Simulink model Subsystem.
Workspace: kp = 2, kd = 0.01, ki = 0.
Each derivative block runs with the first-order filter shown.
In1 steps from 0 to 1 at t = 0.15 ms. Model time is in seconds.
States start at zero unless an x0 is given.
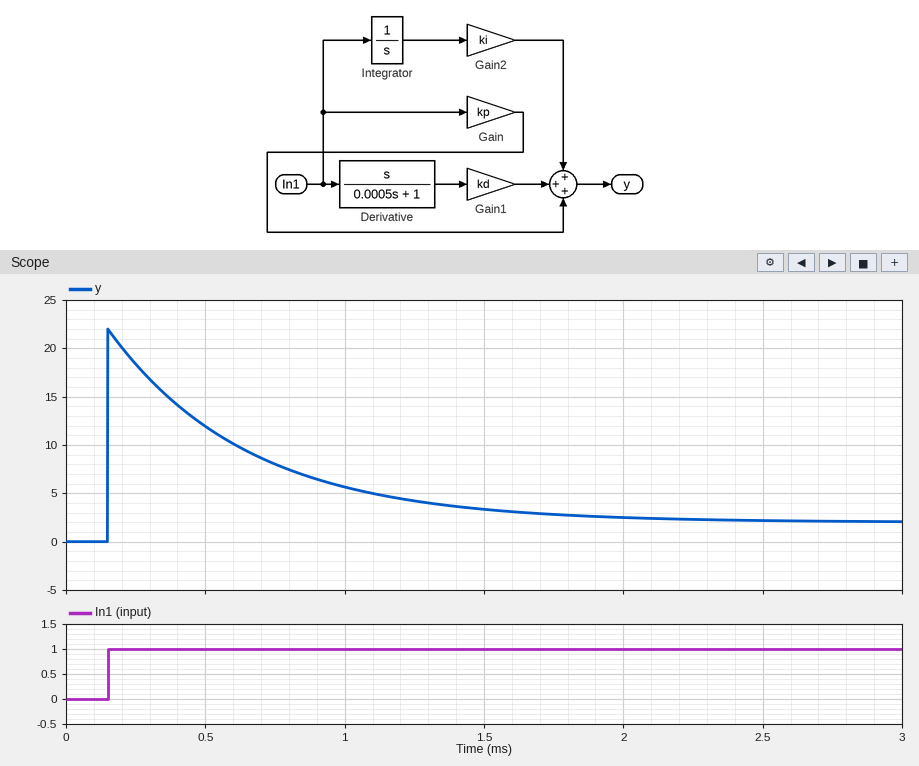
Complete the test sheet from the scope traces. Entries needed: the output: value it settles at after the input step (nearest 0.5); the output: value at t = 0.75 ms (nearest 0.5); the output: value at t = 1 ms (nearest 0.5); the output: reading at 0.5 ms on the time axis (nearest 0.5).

2.0
8.0
5.5
12.0
